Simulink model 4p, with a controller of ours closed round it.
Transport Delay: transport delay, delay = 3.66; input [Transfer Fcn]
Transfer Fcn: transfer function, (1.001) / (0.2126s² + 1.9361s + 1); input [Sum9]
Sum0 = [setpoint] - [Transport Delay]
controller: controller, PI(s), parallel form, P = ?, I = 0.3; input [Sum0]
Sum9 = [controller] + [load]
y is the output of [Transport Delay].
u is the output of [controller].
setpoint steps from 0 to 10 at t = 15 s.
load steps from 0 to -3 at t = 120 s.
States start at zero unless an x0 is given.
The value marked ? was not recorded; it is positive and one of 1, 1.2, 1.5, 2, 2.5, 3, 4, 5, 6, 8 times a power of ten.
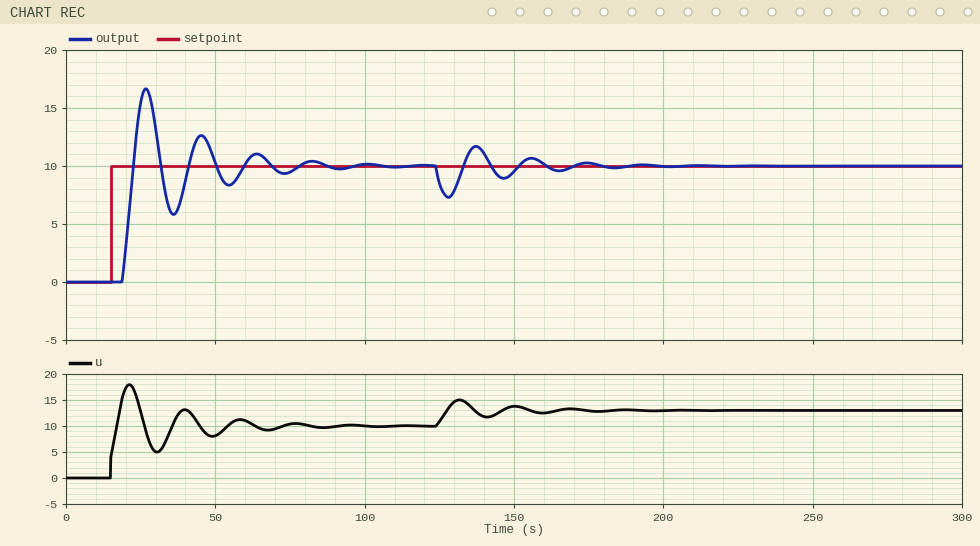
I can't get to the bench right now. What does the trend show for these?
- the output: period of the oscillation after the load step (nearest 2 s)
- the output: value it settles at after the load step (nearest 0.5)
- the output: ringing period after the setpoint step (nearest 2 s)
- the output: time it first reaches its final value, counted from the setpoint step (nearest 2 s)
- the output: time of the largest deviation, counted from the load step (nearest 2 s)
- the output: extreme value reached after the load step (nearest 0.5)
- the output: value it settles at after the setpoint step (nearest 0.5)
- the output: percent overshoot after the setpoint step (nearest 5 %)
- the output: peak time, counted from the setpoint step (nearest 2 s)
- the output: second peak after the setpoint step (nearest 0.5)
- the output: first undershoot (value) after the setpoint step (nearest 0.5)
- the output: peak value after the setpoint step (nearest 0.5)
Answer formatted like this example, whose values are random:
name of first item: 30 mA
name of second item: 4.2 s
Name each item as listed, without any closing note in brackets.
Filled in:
the output: period of the oscillation after the load step: 18 s
the output: value it settles at after the load step: 10.0
the output: ringing period after the setpoint step: 18 s
the output: time it first reaches its final value, counted from the setpoint step: 8 s
the output: time of the largest deviation, counted from the load step: 8 s
the output: extreme value reached after the load step: 7.5
the output: value it settles at after the setpoint step: 10.0
the output: percent overshoot after the setpoint step: 65 %
the output: peak time, counted from the setpoint step: 12 s
the output: second peak after the setpoint step: 12.5
the output: first undershoot (value) after the setpoint step: 6.0
the output: peak value after the setpoint step: 16.5
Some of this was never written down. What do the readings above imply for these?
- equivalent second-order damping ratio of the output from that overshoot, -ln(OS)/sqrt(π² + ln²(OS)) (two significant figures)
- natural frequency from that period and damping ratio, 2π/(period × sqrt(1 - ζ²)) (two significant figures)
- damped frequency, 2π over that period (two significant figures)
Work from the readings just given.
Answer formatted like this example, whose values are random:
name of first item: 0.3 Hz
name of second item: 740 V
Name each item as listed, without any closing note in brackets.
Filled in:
equivalent second-order damping ratio of the output from that overshoot, -ln(OS)/sqrt(π² + ln²(OS)): 0.14
natural frequency from that period and damping ratio, 2π/(period × sqrt(1 - ζ²)): 0.35 rad/s
damped frequency, 2π over that period: 0.35 rad/s
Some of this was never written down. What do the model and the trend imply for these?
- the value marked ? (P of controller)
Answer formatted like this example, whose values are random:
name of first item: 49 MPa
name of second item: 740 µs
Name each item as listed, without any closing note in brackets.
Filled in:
the value marked ?: 0.4
